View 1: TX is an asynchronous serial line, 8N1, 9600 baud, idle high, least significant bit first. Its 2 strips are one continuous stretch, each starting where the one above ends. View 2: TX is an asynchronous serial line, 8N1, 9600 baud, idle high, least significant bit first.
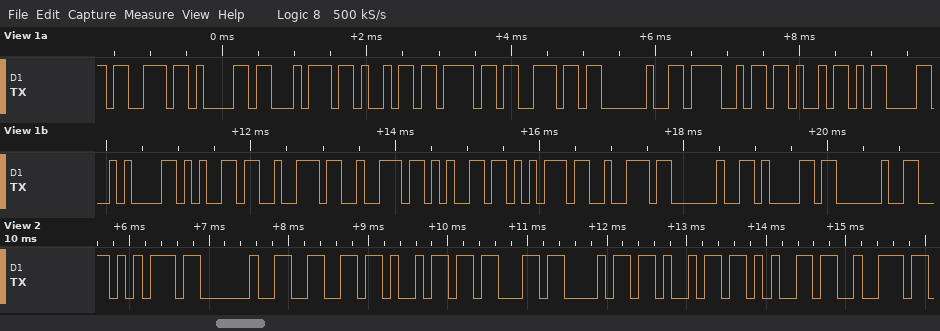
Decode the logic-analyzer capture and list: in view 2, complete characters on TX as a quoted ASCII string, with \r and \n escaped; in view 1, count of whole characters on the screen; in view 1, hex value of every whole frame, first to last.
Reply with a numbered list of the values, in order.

1. "u fichier"
2. 20
3. 73 61 74 69 6F 6E 20 4F 4B 0D 0A 65 72 72 65 75 72 20 61 20
